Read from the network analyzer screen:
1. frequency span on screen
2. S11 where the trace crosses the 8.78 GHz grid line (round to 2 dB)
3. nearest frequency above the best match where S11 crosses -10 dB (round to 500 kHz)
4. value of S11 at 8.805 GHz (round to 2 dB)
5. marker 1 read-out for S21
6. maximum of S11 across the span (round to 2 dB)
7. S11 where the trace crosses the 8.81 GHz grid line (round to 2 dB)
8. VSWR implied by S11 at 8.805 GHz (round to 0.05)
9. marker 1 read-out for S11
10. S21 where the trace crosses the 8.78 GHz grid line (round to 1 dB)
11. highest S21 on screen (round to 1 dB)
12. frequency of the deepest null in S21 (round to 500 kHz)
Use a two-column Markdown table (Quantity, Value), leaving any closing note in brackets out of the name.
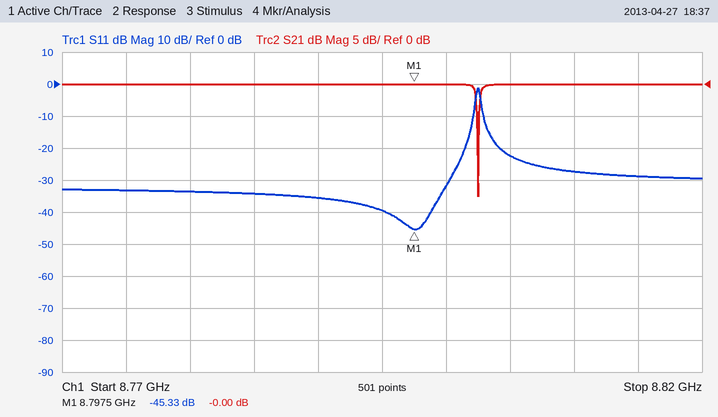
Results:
| Quantity | Value |
|---|---|
| frequency span on screen | 50 MHz |
| S11 where the trace crosses the 8.78 GHz grid line | -34 dB |
| nearest frequency above the best match where S11 crosses -10 dB | 8.8020 GHz |
| value of S11 at 8.805 GHz | -22 dB |
| marker 1 read-out for S21 | -0.00 dB |
| maximum of S11 across the span | -2 dB |
| S11 where the trace crosses the 8.81 GHz grid line | -28 dB |
| VSWR implied by S11 at 8.805 GHz | 1.15 |
| marker 1 read-out for S11 | -45.33 dB |
| S21 where the trace crosses the 8.78 GHz grid line | 0 dB |
| highest S21 on screen | 0 dB |
| frequency of the deepest null in S21 | 8.8025 GHz |
